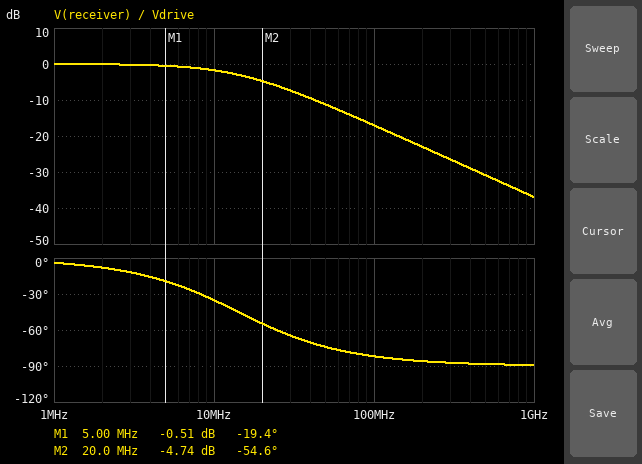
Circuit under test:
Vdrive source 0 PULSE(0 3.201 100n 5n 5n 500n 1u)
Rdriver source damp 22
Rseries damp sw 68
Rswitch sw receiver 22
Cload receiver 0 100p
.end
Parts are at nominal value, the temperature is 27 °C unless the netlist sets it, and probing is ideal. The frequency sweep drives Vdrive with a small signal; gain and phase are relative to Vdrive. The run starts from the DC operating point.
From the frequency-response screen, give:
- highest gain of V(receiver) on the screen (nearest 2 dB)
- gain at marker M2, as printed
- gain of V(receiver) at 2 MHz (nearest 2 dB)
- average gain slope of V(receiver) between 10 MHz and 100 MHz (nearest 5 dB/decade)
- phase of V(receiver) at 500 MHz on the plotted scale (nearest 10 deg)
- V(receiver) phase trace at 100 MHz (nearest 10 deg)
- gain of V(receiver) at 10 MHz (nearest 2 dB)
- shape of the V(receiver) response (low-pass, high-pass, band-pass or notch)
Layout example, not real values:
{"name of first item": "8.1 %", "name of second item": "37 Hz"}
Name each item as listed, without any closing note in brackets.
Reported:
{"highest gain of V(receiver) on the screen": "0 dB", "gain at marker M2, as printed": "-4.74 dB", "gain of V(receiver) at 2 MHz": "0 dB", "average gain slope of V(receiver) between 10 MHz and 100 MHz": "-15 dB/decade", "phase of V(receiver) at 500 MHz on the plotted scale": "-90 deg", "V(receiver) phase trace at 100 MHz": "-80 deg", "gain of V(receiver) at 10 MHz": "-2 dB", "shape of the V(receiver) response": "low-pass"}
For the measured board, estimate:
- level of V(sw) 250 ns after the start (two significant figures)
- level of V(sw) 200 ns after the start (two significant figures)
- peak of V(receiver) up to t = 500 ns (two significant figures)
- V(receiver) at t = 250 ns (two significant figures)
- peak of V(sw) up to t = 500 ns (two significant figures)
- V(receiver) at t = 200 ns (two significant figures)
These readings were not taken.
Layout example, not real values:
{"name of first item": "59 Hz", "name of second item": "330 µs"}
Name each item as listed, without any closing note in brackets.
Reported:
{"level of V(sw) 250 ns after the start": "3.2 V", "level of V(sw) 200 ns after the start": "3.2 V", "peak of V(receiver) up to t = 500 ns": "3.2 V", "V(receiver) at t = 250 ns": "3.2 V", "peak of V(sw) up to t = 500 ns": "3.2 V", "V(receiver) at t = 200 ns": "3.2 V"}
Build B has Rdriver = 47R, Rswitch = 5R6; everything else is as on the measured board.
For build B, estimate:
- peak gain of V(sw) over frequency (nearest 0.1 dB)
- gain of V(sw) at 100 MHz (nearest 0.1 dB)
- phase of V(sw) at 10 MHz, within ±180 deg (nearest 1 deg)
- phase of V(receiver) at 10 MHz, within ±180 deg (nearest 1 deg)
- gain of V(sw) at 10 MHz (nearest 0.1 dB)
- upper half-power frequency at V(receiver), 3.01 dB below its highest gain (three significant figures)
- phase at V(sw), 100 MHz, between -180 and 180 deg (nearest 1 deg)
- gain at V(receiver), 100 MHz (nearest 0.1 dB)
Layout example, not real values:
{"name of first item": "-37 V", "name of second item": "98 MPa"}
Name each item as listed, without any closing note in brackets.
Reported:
{"peak gain of V(sw) over frequency": "0 dB", "gain of V(sw) at 100 MHz": "-17.2 dB", "phase of V(sw) at 10 MHz, within ±180 deg": "-35 deg", "phase of V(receiver) at 10 MHz, within ±180 deg": "-37 deg", "gain of V(sw) at 10 MHz": "-2.0 dB", "upper half-power frequency at V(receiver), 3.01 dB below its highest gain": "13.2 MHz", "phase at V(sw), 100 MHz, between -180 and 180 deg": "-63 deg", "gain at V(receiver), 100 MHz": "-17.7 dB"}
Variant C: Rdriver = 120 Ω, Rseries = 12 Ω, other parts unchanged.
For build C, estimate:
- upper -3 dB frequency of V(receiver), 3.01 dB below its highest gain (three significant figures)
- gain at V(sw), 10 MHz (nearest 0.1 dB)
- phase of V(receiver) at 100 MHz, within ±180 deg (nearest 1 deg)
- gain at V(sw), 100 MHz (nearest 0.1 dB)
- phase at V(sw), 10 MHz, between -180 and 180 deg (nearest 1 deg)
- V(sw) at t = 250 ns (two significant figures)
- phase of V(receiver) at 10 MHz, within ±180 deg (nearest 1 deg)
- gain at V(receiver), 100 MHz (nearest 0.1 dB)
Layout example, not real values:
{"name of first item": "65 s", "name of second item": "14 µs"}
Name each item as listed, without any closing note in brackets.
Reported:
{"upper -3 dB frequency of V(receiver), 3.01 dB below its highest gain": "10.3 MHz", "gain at V(sw), 10 MHz": "-2.8 dB", "phase of V(receiver) at 100 MHz, within ±180 deg": "-84 deg", "gain at V(sw), 100 MHz": "-15.1 dB", "phase at V(sw), 10 MHz, between -180 and 180 deg": "-36 deg", "V(sw) at t = 250 ns": "3.2 V", "phase of V(receiver) at 10 MHz, within ±180 deg": "-44 deg", "gain at V(receiver), 100 MHz": "-19.8 dB"}
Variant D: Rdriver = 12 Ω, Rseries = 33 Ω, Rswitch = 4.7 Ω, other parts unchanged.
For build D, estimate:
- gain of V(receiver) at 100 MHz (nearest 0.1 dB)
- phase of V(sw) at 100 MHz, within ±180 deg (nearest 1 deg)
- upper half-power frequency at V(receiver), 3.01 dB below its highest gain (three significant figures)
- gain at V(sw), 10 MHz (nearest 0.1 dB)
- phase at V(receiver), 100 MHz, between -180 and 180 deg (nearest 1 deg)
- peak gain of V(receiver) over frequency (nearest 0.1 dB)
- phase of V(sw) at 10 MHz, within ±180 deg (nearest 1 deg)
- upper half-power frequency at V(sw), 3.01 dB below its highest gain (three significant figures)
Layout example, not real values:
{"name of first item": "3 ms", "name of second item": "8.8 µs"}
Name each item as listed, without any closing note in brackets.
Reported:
{"gain of V(receiver) at 100 MHz": "-10.3 dB", "phase of V(sw) at 100 MHz, within ±180 deg": "-56 deg", "upper half-power frequency at V(receiver), 3.01 dB below its highest gain": "32.0 MHz", "gain at V(sw), 10 MHz": "-0.4 dB", "phase at V(receiver), 100 MHz, between -180 and 180 deg": "-72 deg", "peak gain of V(receiver) over frequency": "0 dB", "phase of V(sw) at 10 MHz, within ±180 deg": "-16 deg", "upper half-power frequency at V(sw), 3.01 dB below its highest gain": "32.3 MHz"}
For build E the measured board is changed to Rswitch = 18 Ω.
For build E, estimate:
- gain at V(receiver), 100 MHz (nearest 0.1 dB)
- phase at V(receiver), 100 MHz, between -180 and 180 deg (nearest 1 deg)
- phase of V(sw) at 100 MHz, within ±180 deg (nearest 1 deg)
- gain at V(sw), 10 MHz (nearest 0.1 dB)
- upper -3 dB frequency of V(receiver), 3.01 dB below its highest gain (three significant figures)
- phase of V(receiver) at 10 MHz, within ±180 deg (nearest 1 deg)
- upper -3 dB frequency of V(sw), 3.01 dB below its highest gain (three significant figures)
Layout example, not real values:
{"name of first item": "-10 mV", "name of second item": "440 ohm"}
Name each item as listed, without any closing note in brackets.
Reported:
{"gain at V(receiver), 100 MHz": "-16.7 dB", "phase at V(receiver), 100 MHz, between -180 and 180 deg": "-82 deg", "phase of V(sw) at 100 MHz, within ±180 deg": "-33 deg", "gain at V(sw), 10 MHz": "-1.6 dB", "upper -3 dB frequency of V(receiver), 3.01 dB below its highest gain": "14.7 MHz", "phase of V(receiver) at 10 MHz, within ±180 deg": "-34 deg", "upper -3 dB frequency of V(sw), 3.01 dB below its highest gain": "15.2 MHz"}
